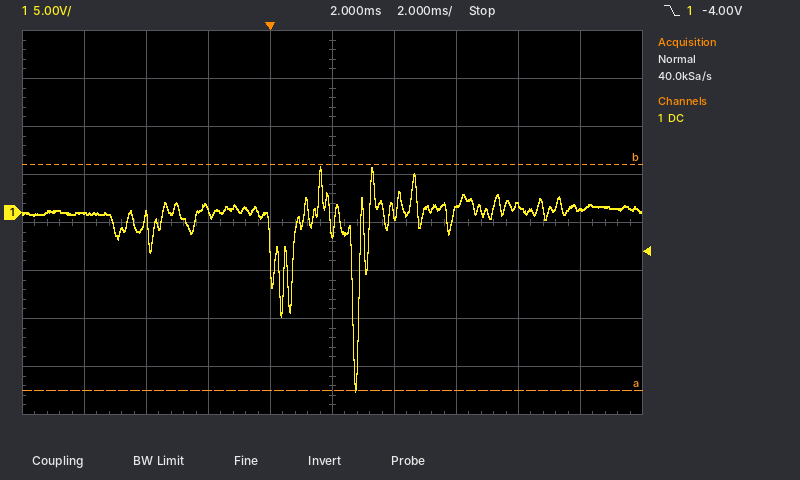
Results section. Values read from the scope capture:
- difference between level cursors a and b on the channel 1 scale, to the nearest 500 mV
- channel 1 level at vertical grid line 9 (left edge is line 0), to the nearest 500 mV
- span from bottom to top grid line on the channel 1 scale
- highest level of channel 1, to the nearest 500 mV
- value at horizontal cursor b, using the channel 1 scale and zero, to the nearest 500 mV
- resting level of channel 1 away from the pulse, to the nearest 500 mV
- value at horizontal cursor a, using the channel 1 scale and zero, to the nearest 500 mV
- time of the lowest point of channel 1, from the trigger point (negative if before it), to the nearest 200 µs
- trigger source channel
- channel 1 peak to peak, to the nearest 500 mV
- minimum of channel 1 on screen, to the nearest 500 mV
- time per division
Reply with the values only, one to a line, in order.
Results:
23.5 V
500 mV
40 V
5.0 V
5.0 V
0.0 V
-18.5 V
+2.8 ms
channel 1
23.5 V
-18.5 V
2 ms
